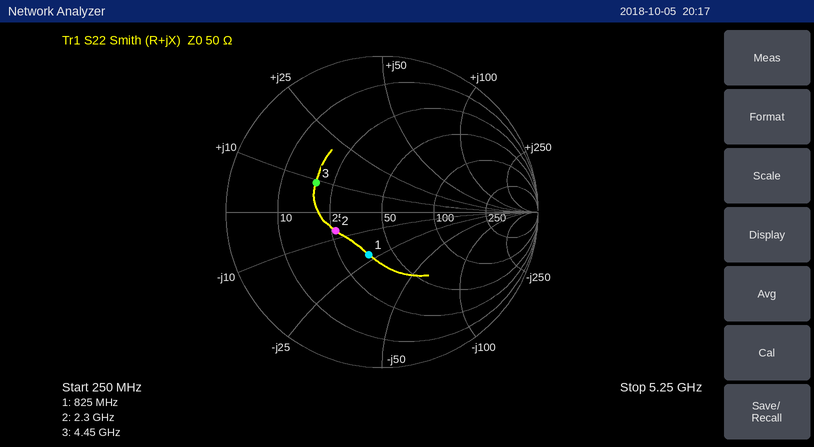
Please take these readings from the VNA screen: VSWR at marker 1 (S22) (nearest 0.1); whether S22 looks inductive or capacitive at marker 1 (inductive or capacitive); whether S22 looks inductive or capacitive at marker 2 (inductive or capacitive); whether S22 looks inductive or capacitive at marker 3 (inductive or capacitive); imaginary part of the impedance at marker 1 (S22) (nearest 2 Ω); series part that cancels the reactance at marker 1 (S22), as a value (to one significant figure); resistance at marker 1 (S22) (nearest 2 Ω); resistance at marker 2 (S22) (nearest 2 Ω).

1.8
capacitive
capacitive
inductive
-22 Ω
4 nH
36 Ω
26 Ω
